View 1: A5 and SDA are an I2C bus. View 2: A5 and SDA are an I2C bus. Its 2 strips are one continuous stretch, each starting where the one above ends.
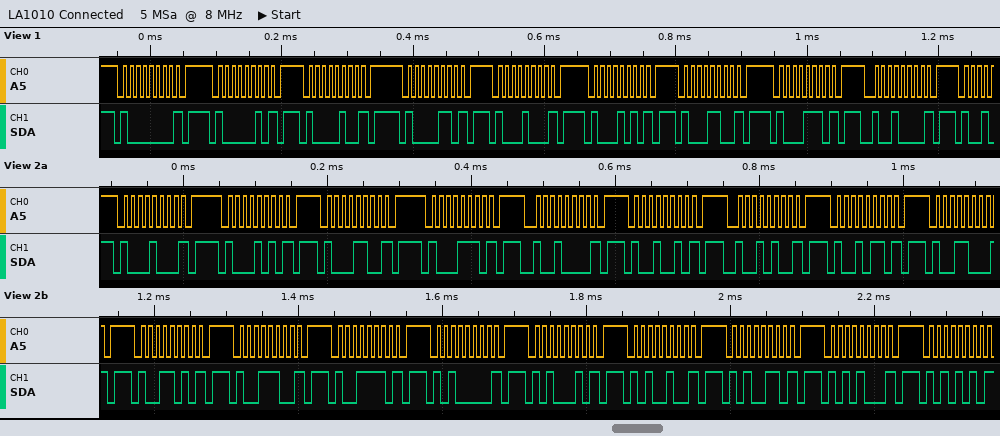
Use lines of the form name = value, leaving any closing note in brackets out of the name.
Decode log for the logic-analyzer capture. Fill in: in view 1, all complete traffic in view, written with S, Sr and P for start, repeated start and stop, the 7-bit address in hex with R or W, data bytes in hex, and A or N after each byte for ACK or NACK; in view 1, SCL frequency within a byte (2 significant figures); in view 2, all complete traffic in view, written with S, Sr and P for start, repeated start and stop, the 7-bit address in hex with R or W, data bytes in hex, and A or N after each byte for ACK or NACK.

in view 1, all complete traffic in view, written with S, Sr and P for start, repeated start and stop, the 7-bit address in hex with R or W, data bytes in hex, and A or N after each byte for ACK or NACK = S 40W N P S 41W N P S 42W N P S 43W N P S 44W N P S 45W N P S 46W N P S 47W N P S 48W N P
in view 1, SCL frequency within a byte = 100 kHz
in view 2, all complete traffic in view, written with S, Sr and P for start, repeated start and stop, the 7-bit address in hex with R or W, data bytes in hex, and A or N after each byte for ACK or NACK = S 44W N P S 45W N P S 46W N P S 47W N P S 48W N P S 49W N P S 4AW N P S 4BW N P S 4CW N P S 4DW N P S 4EW N P S 4FW N P S 50W N P S 51W N P S 52W N P S 53W N P S 54W N P S 55W N
